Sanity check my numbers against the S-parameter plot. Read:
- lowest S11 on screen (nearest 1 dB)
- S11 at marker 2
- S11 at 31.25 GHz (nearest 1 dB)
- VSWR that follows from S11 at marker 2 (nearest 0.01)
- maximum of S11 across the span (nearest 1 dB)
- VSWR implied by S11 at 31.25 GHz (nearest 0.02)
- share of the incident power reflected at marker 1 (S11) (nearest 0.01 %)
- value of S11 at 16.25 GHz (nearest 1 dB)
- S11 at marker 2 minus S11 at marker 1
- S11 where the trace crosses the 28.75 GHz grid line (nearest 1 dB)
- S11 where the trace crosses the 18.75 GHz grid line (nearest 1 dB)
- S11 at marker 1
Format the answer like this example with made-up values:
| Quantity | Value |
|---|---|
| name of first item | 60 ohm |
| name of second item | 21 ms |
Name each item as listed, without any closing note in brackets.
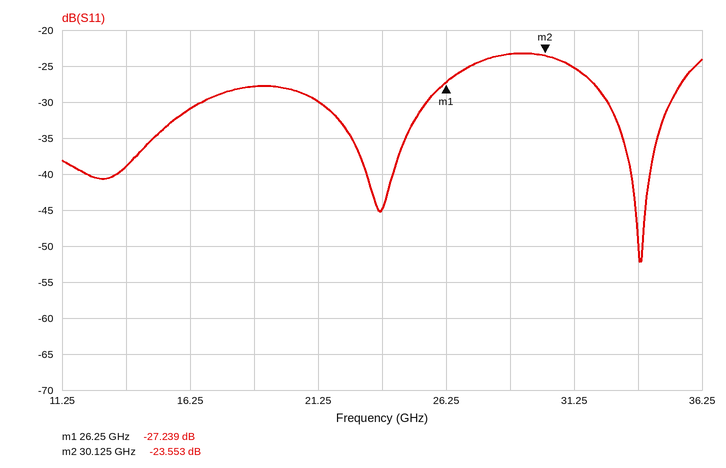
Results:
| Quantity | Value |
|---|---|
| lowest S11 on screen | -52 dB |
| S11 at marker 2 | -23.553 dB |
| S11 at 31.25 GHz | -25 dB |
| VSWR that follows from S11 at marker 2 | 1.14 |
| maximum of S11 across the span | -23 dB |
| VSWR implied by S11 at 31.25 GHz | 1.12 |
| share of the incident power reflected at marker 1 (S11) | 0.19 % |
| value of S11 at 16.25 GHz | -31 dB |
| S11 at marker 2 minus S11 at marker 1 | 3.686 dB |
| S11 where the trace crosses the 28.75 GHz grid line | -23 dB |
| S11 where the trace crosses the 18.75 GHz grid line | -28 dB |
| S11 at marker 1 | -27.239 dB |
